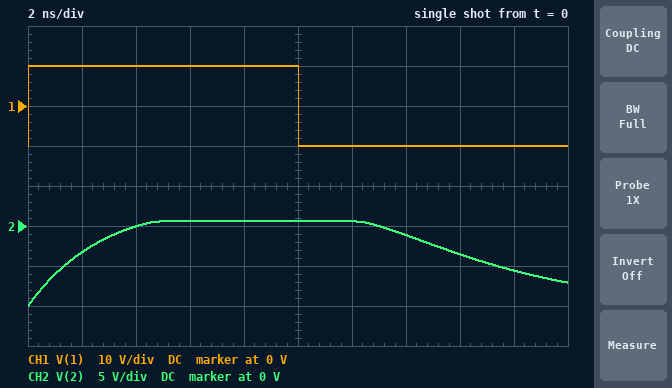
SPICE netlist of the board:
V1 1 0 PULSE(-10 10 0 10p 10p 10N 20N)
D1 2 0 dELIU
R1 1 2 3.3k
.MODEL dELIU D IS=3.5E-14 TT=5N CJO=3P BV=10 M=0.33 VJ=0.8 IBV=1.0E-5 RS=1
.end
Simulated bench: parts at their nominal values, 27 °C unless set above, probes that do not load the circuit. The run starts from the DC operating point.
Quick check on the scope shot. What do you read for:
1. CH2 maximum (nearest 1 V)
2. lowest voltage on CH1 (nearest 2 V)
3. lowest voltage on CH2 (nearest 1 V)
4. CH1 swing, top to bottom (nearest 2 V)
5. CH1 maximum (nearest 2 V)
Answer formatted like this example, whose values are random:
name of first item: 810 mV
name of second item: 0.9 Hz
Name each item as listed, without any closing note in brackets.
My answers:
CH2 maximum: 1 V
lowest voltage on CH1: -10 V
lowest voltage on CH2: -10 V
CH1 swing, top to bottom: 20 V
CH1 maximum: 10 V
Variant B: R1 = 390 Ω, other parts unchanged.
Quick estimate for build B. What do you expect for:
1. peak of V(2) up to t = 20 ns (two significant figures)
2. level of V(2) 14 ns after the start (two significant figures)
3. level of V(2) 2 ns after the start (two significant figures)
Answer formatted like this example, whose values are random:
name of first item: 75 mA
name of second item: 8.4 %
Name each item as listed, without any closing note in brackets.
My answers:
peak of V(2) up to t = 20 ns: 720 mV
level of V(2) 14 ns after the start: -8.3 V
level of V(2) 2 ns after the start: 690 mV
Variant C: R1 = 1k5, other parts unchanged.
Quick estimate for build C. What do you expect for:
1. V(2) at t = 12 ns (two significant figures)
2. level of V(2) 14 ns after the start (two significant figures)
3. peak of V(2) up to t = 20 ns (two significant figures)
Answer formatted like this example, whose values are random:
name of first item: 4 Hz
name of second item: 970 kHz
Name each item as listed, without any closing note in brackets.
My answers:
V(2) at t = 12 ns: 620 mV
level of V(2) 14 ns after the start: -2.6 V
peak of V(2) up to t = 20 ns: 670 mV
